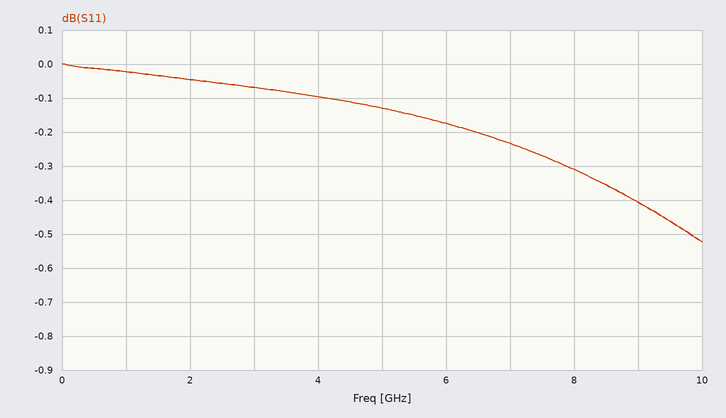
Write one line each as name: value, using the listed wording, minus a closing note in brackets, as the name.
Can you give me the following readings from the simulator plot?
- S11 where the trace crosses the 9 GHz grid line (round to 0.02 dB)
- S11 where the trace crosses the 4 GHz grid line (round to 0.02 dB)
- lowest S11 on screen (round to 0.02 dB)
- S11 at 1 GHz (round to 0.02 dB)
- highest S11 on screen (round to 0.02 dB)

S11 where the trace crosses the 9 GHz grid line: -0.40 dB
S11 where the trace crosses the 4 GHz grid line: -0.10 dB
lowest S11 on screen: -0.52 dB
S11 at 1 GHz: -0.02 dB
highest S11 on screen: 0.00 dB
